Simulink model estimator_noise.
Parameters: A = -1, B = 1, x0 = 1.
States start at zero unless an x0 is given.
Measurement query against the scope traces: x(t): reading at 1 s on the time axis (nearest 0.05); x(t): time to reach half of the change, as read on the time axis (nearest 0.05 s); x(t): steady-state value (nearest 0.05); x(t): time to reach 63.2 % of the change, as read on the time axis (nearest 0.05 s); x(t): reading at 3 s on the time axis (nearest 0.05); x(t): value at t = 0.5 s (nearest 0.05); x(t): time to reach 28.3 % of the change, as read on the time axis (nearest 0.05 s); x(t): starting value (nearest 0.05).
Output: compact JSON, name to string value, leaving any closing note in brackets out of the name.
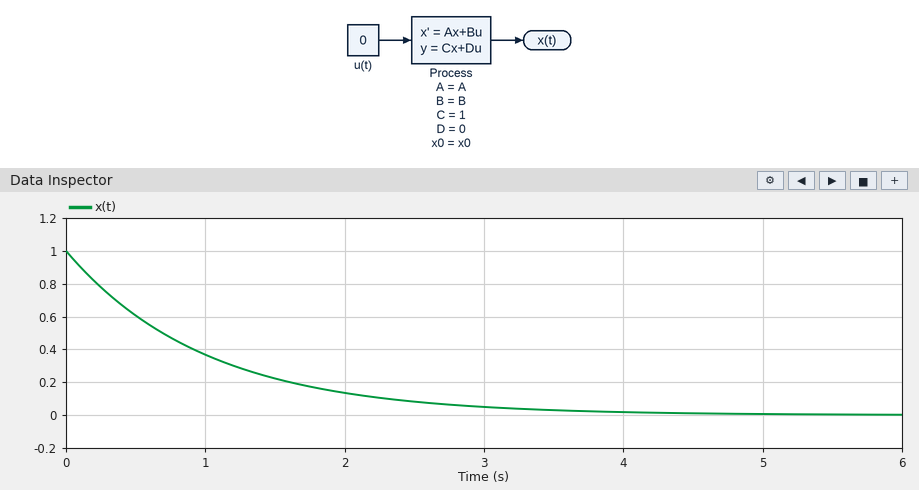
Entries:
{"x(t): reading at 1 s on the time axis": "0.35", "x(t): time to reach half of the change, as read on the time axis": "0.70 s", "x(t): steady-state value": "0.00", "x(t): time to reach 63.2 % of the change, as read on the time axis": "1.00 s", "x(t): reading at 3 s on the time axis": "0.05", "x(t): value at t = 0.5 s": "0.60", "x(t): time to reach 28.3 % of the change, as read on the time axis": "0.35 s", "x(t): starting value": "1.00"}
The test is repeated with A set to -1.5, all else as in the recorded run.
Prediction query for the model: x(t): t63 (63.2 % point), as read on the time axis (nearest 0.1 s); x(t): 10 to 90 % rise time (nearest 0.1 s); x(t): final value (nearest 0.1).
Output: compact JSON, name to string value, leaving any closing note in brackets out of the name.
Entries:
{"x(t): t63 (63.2 % point), as read on the time axis": "0.7 s", "x(t): 10 to 90 % rise time": "1.5 s", "x(t): final value": "0.0"}
